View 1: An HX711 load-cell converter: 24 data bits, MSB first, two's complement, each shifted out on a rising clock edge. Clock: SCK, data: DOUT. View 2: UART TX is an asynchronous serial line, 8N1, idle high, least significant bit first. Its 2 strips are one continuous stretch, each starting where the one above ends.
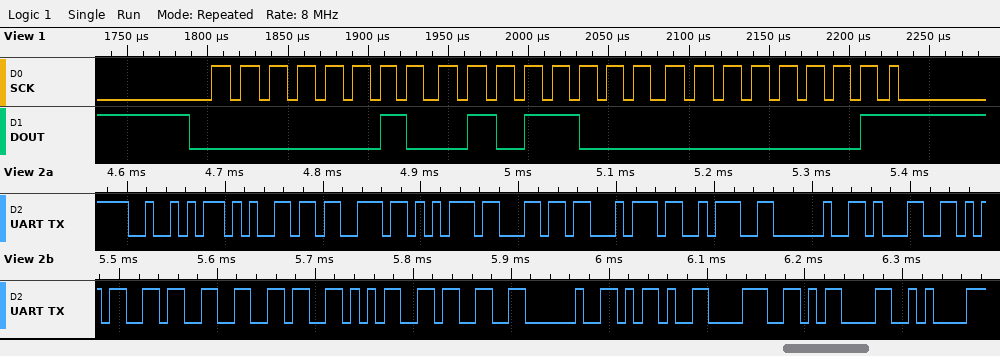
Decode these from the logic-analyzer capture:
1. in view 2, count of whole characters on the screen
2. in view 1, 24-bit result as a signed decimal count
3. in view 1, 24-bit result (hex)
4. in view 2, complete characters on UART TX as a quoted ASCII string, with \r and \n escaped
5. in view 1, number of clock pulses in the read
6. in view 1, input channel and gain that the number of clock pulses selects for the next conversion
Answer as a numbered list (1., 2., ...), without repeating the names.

1. 19
2. 153601
3. 0x025801
4. "Result: 153653 -8\r\n"
5. 25
6. channel A, gain 128
